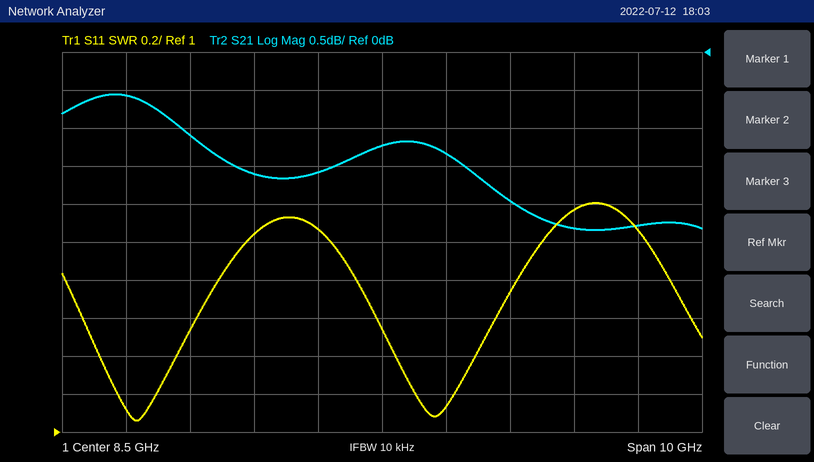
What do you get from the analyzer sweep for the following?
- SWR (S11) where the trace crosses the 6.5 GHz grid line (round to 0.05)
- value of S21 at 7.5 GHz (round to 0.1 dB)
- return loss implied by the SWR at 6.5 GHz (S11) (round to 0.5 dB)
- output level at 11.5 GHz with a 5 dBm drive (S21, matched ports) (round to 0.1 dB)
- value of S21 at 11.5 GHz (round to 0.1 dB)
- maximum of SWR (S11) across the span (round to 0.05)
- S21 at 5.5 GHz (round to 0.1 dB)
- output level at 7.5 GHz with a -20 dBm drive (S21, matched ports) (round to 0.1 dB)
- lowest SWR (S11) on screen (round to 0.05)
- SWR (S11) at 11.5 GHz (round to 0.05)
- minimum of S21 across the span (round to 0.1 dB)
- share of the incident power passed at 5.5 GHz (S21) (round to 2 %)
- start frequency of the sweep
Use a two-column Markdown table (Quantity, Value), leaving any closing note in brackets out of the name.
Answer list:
| Quantity | Value |
|---|---|
| SWR (S11) where the trace crosses the 6.5 GHz grid line | 2.05 |
| value of S21 at 7.5 GHz | -1.6 dB |
| return loss implied by the SWR at 6.5 GHz (S11) | 9.5 dB |
| output level at 11.5 GHz with a 5 dBm drive (S21, matched ports) | 2.7 dBm |
| value of S21 at 11.5 GHz | -2.3 dB |
| maximum of SWR (S11) across the span | 2.20 |
| S21 at 5.5 GHz | -1.1 dB |
| output level at 7.5 GHz with a -20 dBm drive (S21, matched ports) | -21.6 dBm |
| lowest SWR (S11) on screen | 1.05 |
| SWR (S11) at 11.5 GHz | 2.15 |
| minimum of S21 across the span | -2.3 dB |
| share of the incident power passed at 5.5 GHz (S21) | 78 % |
| start frequency of the sweep | 3.5 GHz |
